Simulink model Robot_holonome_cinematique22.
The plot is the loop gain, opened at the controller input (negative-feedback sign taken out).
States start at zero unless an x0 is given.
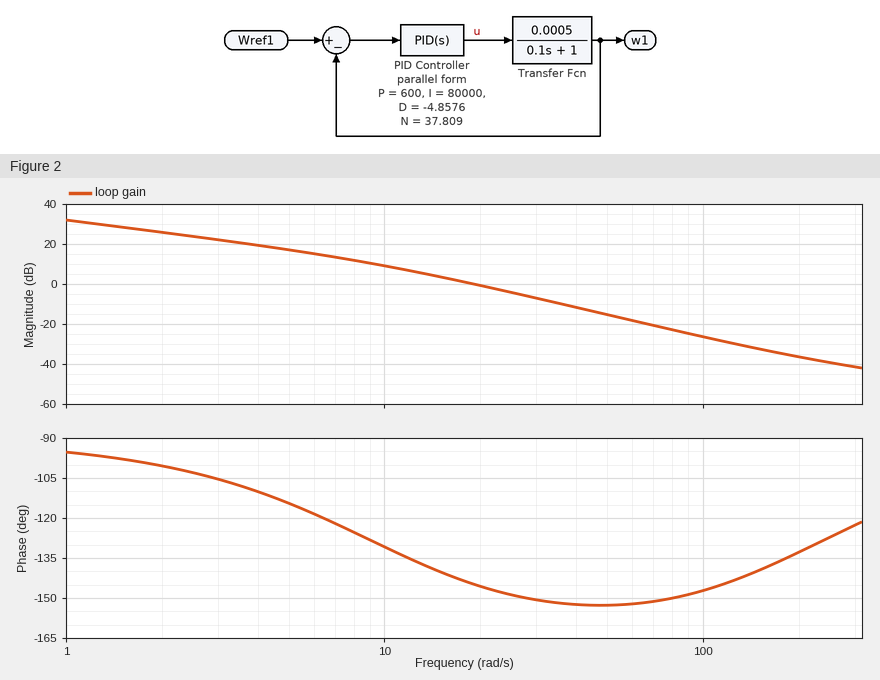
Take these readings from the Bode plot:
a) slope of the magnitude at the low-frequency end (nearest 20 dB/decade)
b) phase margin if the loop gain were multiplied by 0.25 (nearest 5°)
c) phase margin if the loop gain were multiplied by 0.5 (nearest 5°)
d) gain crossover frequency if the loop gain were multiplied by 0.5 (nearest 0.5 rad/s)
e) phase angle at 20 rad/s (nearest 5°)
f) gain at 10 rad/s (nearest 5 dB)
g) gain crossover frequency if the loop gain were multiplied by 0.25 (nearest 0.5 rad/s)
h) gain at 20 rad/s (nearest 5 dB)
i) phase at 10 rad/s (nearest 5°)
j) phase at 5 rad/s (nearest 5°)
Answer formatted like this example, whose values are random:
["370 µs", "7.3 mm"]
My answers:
["-20 dB/decade", "55°", "45°", "12.5 rad/s", "-145°", "10 dB", "8.0 rad/s", "0 dB", "-130°", "-115°"]
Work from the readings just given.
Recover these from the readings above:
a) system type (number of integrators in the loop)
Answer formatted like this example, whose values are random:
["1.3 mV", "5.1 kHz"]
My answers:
["1"]
